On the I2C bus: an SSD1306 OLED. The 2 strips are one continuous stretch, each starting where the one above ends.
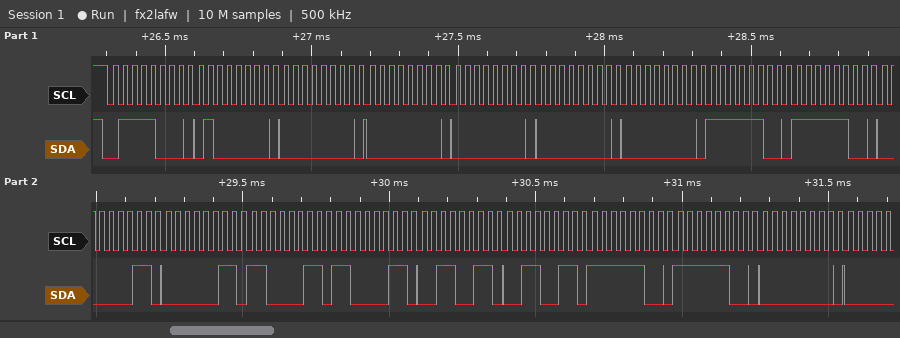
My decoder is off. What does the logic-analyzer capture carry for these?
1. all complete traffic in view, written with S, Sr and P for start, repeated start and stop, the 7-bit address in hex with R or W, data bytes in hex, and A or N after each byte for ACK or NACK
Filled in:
S 3CW A 40 A 00 A 00 A 00 A 00 A 00 A FC A FC A 03 A 03 A C3 A C3 A 33 A 33 A FC A FC A 00 A
